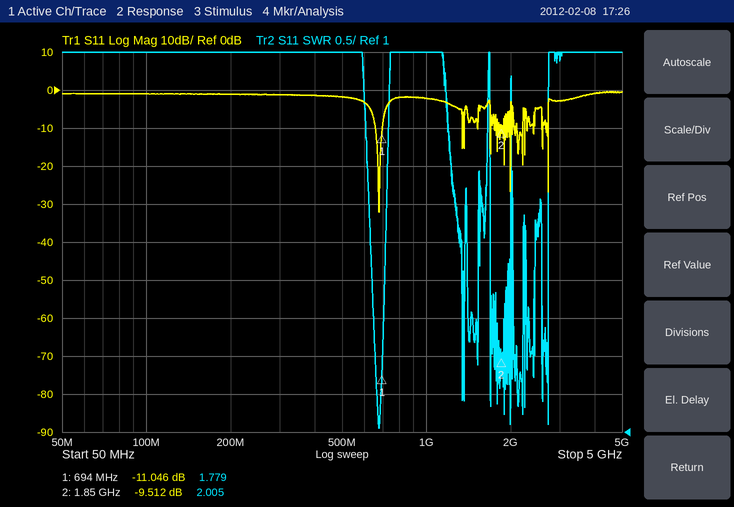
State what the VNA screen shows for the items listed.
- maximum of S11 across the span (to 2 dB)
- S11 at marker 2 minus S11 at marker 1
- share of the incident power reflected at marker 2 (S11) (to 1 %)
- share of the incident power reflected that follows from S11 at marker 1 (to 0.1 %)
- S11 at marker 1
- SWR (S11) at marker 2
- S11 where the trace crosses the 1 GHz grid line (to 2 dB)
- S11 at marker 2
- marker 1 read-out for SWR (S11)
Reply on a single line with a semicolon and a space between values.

0 dB; 1.534 dB; 11 %; 7.9 %; -11.046 dB; 2.005; -2 dB; -9.512 dB; 1.779
